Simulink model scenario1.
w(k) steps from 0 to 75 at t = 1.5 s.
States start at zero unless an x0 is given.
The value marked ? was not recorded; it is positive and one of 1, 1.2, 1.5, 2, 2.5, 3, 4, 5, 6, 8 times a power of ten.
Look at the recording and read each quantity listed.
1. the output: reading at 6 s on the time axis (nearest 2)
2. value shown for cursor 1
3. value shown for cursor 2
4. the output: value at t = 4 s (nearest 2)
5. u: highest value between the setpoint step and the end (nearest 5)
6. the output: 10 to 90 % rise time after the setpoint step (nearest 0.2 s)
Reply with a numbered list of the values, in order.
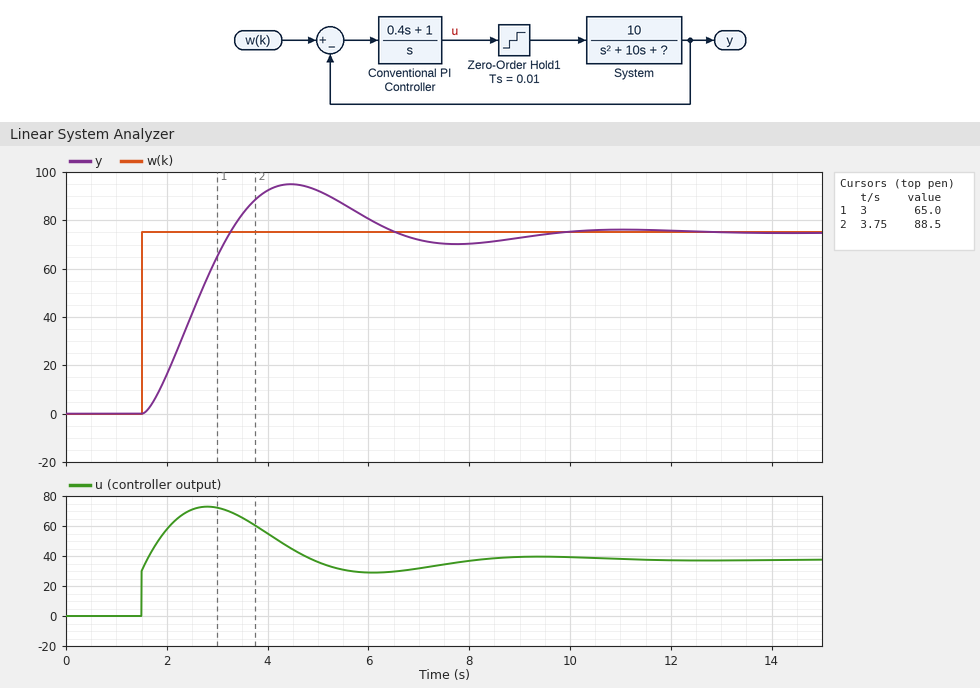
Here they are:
1. 80
2. 65.0
3. 88.5
4. 92
5. 75
6. 1.2 s
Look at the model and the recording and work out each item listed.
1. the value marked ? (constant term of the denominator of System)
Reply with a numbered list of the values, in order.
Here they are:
1. 5
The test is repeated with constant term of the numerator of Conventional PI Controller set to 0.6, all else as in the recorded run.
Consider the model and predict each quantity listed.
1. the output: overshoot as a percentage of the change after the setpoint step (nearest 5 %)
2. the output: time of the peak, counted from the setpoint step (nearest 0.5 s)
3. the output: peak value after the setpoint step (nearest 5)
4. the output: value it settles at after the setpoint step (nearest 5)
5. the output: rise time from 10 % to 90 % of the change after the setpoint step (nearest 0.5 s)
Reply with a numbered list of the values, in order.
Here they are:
1. 15 %
2. 4.0 s
3. 85
4. 75
5. 2.0 s
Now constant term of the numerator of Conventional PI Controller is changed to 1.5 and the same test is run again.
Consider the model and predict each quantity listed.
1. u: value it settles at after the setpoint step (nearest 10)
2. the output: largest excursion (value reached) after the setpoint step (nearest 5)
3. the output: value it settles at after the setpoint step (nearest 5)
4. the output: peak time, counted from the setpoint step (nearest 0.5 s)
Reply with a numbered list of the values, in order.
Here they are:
1. 40
2. 105
3. 75
4. 2.5 s
